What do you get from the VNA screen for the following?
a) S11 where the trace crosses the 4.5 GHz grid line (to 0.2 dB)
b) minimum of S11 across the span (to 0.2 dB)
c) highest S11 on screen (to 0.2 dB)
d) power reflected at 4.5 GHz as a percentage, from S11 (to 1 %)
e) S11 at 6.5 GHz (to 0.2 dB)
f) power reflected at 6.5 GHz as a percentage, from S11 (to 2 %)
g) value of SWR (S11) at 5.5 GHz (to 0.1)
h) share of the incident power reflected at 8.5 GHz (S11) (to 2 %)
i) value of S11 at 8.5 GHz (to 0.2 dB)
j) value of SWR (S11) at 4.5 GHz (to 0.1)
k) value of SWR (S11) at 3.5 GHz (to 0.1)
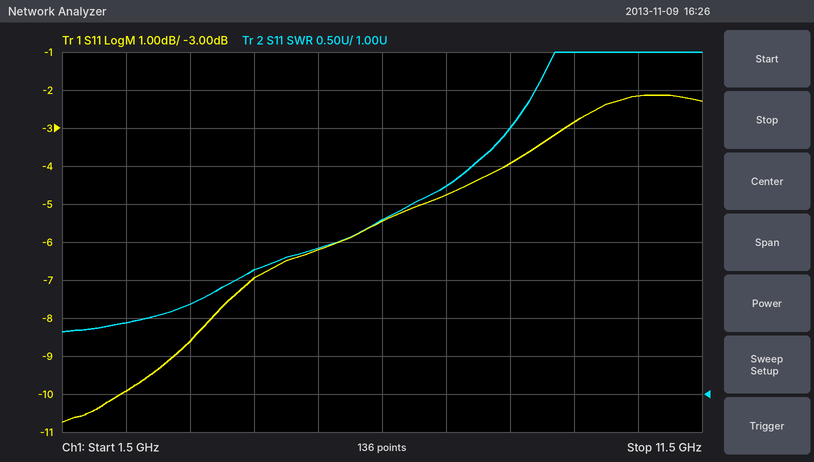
-7.0 dB
-10.8 dB
-2.2 dB
20 %
-5.4 dB
28 %
2.9
40 %
-4.0 dB
2.6
2.2
